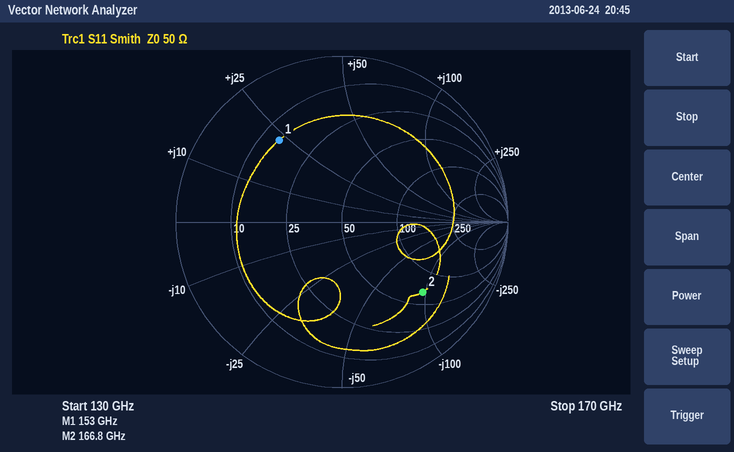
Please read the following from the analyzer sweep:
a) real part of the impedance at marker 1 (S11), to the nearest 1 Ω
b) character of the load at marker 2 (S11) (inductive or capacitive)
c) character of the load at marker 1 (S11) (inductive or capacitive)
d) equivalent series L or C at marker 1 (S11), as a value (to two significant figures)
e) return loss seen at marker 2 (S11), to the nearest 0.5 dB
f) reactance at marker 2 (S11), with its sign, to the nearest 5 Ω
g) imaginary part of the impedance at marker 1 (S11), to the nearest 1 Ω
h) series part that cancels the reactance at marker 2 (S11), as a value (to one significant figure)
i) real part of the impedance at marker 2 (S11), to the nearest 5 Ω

14 Ω
capacitive
inductive
24 pH
4.0 dB
-95 Ω
+23 Ω
90 pH
65 Ω
